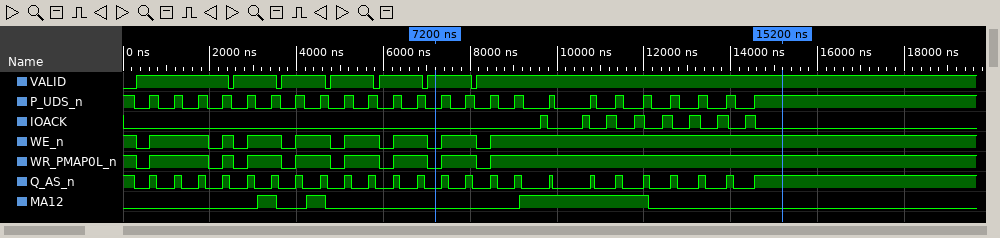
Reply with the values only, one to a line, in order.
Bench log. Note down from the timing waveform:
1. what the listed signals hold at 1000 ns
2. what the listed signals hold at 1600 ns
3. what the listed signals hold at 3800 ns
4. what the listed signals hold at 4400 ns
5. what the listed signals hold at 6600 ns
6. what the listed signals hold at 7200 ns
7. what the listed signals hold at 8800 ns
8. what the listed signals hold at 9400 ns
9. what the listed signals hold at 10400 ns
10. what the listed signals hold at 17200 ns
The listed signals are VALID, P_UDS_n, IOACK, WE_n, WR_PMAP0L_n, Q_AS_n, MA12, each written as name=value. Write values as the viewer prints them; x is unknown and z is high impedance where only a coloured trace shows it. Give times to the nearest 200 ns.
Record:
VALID=1, P_UDS_n=0, IOACK=0, WE_n=1, WR_PMAP0L_n=1, Q_AS_n=0, MA12=0
VALID=1, P_UDS_n=0, IOACK=0, WE_n=1, WR_PMAP0L_n=1, Q_AS_n=0, MA12=0
VALID=1, P_UDS_n=0, IOACK=0, WE_n=0, WR_PMAP0L_n=0, Q_AS_n=0, MA12=0
VALID=1, P_UDS_n=0, IOACK=0, WE_n=1, WR_PMAP0L_n=1, Q_AS_n=0, MA12=1
VALID=1, P_UDS_n=0, IOACK=0, WE_n=1, WR_PMAP0L_n=1, Q_AS_n=0, MA12=0
VALID=1, P_UDS_n=0, IOACK=0, WE_n=0, WR_PMAP0L_n=0, Q_AS_n=0, MA12=0
VALID=1, P_UDS_n=0, IOACK=0, WE_n=1, WR_PMAP0L_n=1, Q_AS_n=0, MA12=0
VALID=1, P_UDS_n=0, IOACK=0, WE_n=1, WR_PMAP0L_n=1, Q_AS_n=0, MA12=1
VALID=1, P_UDS_n=0, IOACK=0, WE_n=1, WR_PMAP0L_n=1, Q_AS_n=0, MA12=1
VALID=1, P_UDS_n=1, IOACK=0, WE_n=1, WR_PMAP0L_n=1, Q_AS_n=1, MA12=0
